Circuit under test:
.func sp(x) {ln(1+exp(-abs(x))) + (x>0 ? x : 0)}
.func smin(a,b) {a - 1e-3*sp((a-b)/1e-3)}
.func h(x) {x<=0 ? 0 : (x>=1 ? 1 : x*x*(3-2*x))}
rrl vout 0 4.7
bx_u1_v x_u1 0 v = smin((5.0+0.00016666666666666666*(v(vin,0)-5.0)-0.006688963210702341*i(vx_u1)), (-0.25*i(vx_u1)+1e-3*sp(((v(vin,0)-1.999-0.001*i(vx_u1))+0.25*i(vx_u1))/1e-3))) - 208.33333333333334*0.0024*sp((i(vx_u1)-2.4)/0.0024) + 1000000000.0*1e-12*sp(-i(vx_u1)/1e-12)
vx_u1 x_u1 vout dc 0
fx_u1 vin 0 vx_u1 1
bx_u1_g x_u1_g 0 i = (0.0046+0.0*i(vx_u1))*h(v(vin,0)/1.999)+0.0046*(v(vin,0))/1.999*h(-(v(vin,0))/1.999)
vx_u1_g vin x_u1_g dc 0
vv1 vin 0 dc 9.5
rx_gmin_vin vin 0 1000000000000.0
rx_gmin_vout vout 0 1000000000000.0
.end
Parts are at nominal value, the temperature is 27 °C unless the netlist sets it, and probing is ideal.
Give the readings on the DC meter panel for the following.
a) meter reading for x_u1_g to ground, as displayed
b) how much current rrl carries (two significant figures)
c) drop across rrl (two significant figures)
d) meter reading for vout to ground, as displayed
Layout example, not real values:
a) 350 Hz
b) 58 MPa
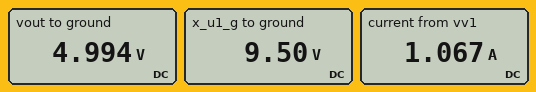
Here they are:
a) 9.50 V
b) 1.1 A
c) 5.0 V
d) 4.994 V
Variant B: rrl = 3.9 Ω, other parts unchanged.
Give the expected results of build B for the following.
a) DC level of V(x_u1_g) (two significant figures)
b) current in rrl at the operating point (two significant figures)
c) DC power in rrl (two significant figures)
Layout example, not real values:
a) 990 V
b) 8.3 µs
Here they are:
a) 9.5 V
b) 1.3 A
c) 6.4 W
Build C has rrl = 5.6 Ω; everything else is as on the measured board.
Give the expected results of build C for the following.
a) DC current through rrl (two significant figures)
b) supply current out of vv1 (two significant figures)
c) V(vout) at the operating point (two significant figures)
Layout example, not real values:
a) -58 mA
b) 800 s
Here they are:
a) 890 mA
b) 900 mA
c) 5.0 V
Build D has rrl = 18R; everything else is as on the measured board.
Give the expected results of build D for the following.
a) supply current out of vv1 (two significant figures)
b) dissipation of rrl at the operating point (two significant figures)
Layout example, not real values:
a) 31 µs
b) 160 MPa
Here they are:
a) 280 mA
b) 1.4 W
